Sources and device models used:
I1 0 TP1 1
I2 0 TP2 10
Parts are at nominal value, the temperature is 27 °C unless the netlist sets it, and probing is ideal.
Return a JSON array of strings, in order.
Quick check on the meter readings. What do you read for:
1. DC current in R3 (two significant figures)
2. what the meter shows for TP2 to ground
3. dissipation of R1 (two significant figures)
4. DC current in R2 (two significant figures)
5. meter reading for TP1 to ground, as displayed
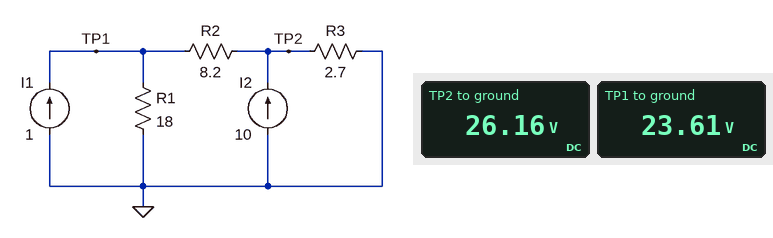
["9.7 A", "26.16 V", "31 W", "310 mA", "23.61 V"]
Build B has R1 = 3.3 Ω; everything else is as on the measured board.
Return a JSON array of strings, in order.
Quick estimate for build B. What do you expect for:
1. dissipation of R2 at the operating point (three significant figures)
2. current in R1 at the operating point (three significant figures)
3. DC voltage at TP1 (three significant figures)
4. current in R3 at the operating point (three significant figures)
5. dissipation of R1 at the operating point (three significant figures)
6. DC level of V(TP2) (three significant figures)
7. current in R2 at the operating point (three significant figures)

["22.8 W", "2.67 A", "8.81 V", "8.33 A", "23.5 W", "22.5 V", "1.67 A"]
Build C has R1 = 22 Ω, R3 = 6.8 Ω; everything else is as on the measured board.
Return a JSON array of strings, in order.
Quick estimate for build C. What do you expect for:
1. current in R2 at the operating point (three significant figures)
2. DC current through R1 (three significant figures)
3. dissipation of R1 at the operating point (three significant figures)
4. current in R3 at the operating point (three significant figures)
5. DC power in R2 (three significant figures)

["1.24 A", "2.24 A", "111 W", "8.76 A", "12.7 W"]
